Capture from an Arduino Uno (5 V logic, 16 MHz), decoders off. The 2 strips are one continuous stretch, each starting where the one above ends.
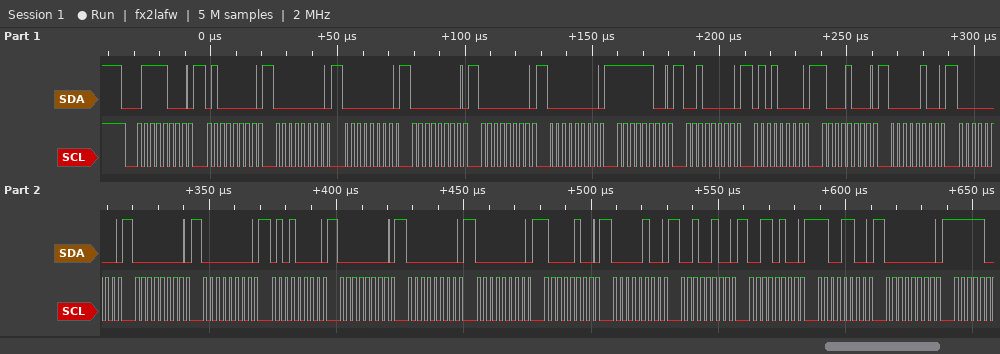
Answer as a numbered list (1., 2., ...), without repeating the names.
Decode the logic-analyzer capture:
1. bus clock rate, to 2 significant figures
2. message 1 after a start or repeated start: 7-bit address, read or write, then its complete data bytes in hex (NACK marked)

1. 400 kHz
2. 0x3C write: 40 00 00 00 00 00 FC 20 50 88 04 00 00 00 50 00 00 00 84 04 24 34 CC 00
